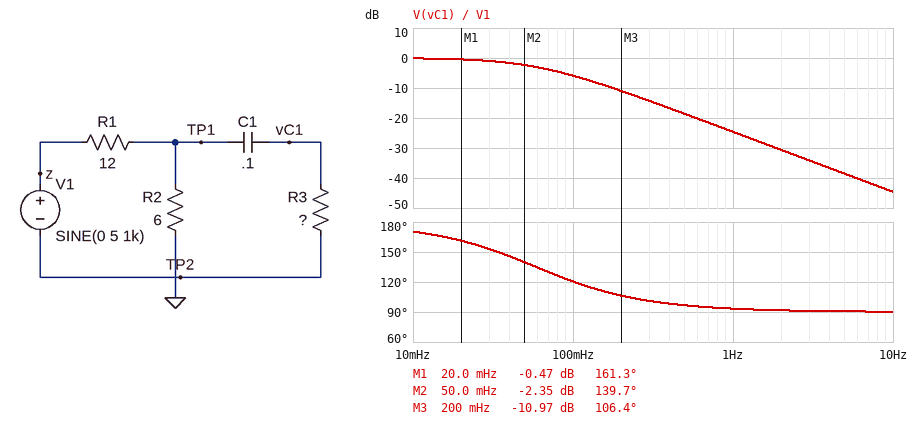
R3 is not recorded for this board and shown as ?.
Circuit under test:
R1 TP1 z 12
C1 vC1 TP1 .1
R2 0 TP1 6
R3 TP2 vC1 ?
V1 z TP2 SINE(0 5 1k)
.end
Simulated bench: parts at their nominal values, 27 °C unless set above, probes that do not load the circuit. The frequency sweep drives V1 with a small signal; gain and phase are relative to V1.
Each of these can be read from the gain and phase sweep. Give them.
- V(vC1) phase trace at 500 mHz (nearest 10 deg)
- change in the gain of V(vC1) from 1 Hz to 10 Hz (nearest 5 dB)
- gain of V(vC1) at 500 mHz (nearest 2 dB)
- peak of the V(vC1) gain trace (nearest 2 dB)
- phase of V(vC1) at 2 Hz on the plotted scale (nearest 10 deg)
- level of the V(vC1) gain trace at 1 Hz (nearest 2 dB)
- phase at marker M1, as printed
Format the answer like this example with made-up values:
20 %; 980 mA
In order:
100 deg; -20 dB; -18 dB; 0 dB; 90 deg; -24 dB; 161.3 deg
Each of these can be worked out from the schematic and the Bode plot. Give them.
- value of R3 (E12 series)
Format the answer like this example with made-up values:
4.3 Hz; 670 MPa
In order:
15 Ω
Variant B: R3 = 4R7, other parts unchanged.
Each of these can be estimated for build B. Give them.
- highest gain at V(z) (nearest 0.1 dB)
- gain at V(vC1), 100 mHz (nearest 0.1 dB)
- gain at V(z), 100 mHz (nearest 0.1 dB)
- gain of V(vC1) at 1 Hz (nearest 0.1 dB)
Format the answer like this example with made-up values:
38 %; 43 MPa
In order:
-2.9 dB; -3.2 dB; -5.7 dB; -20.5 dB
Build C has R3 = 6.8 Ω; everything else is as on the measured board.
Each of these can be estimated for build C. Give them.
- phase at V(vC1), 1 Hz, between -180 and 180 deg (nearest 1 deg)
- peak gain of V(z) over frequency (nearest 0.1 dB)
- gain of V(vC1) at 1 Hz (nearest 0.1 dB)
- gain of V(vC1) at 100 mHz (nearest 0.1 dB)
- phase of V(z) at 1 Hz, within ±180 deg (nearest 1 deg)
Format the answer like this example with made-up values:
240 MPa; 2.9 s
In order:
95 deg; -3.9 dB; -21.5 dB; -3.8 dB; 5 deg
